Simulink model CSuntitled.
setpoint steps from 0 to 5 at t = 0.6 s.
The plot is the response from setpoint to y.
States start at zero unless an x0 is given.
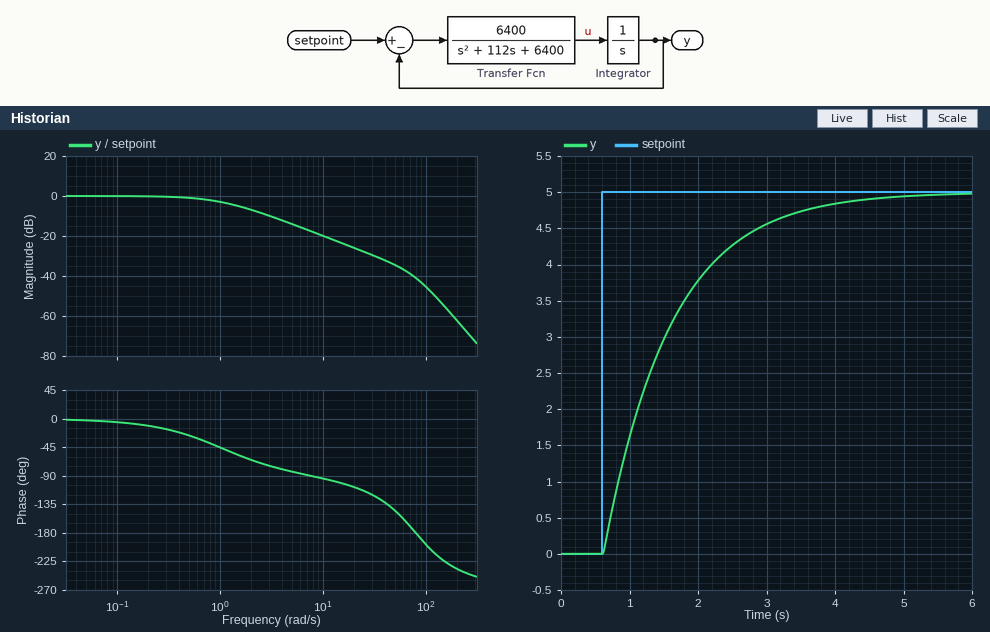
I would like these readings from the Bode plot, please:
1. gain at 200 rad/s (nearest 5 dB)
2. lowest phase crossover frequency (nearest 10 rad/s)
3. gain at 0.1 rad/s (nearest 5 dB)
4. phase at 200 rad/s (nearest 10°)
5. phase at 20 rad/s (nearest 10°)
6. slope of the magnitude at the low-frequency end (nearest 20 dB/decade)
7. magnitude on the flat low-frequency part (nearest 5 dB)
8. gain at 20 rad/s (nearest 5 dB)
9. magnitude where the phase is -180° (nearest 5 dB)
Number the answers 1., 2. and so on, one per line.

1. -60 dB
2. 80 rad/s
3. 0 dB
4. -240°
5. -110°
6. 0 dB/decade
7. 0 dB
8. -25 dB
9. -40 dB
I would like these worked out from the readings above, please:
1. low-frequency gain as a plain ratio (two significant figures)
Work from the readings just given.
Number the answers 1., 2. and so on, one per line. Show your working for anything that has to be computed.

1. 10^(0 / 20) = 1.0
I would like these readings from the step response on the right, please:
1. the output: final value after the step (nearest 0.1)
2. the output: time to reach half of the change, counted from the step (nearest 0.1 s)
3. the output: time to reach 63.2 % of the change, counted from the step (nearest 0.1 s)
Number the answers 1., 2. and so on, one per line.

1. 5.0
2. 0.7 s
3. 1.0 s
